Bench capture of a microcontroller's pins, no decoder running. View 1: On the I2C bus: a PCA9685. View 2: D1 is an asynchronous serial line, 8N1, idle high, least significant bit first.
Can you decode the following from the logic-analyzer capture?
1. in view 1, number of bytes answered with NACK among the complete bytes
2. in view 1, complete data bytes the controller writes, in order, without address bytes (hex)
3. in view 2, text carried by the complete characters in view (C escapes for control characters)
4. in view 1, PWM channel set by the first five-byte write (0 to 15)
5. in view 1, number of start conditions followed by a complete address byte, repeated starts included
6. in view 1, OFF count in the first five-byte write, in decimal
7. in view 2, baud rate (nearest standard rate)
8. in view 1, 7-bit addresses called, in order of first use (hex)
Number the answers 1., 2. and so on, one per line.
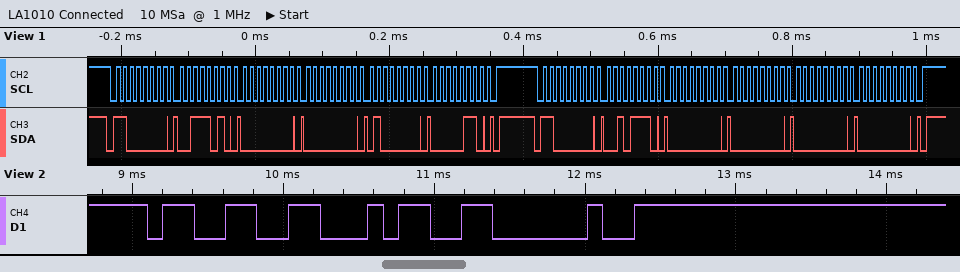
1. 0
2. 3A 00 00 40 06 2E 00 00 00 00
3. "34 "
4. 13
5. 2
6. 1600
7. 9600 baud
8. 0x60
